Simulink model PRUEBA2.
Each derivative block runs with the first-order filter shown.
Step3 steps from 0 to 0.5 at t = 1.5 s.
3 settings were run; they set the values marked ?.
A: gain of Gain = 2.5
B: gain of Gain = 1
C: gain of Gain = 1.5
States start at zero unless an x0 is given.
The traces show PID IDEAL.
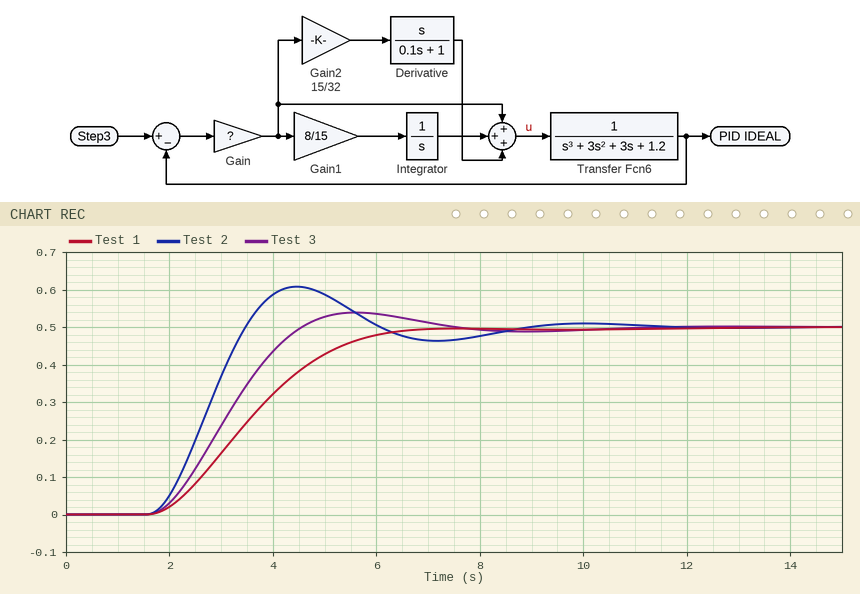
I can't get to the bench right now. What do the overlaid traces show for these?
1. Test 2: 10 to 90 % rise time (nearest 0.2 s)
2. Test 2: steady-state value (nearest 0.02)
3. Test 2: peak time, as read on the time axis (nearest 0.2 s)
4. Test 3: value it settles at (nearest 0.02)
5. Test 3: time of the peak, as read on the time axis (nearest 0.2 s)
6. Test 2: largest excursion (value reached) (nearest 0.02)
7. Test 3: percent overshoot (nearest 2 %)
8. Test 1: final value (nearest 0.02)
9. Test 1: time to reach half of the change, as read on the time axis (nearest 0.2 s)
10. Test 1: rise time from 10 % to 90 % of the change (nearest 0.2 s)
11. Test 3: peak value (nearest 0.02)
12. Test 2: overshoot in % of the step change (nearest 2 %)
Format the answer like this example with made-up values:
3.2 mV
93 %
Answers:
1.2 s
0.50
4.4 s
0.50
5.6 s
0.60
8 %
0.50
3.6 s
3.0 s
0.54
22 %
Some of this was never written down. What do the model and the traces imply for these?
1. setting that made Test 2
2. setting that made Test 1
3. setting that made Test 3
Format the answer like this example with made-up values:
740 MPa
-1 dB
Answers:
A
B
C
